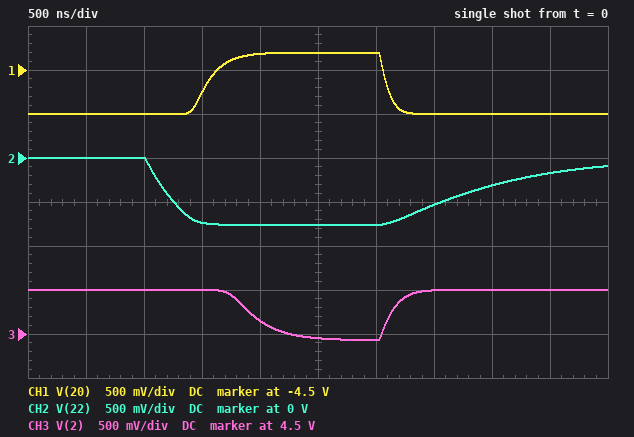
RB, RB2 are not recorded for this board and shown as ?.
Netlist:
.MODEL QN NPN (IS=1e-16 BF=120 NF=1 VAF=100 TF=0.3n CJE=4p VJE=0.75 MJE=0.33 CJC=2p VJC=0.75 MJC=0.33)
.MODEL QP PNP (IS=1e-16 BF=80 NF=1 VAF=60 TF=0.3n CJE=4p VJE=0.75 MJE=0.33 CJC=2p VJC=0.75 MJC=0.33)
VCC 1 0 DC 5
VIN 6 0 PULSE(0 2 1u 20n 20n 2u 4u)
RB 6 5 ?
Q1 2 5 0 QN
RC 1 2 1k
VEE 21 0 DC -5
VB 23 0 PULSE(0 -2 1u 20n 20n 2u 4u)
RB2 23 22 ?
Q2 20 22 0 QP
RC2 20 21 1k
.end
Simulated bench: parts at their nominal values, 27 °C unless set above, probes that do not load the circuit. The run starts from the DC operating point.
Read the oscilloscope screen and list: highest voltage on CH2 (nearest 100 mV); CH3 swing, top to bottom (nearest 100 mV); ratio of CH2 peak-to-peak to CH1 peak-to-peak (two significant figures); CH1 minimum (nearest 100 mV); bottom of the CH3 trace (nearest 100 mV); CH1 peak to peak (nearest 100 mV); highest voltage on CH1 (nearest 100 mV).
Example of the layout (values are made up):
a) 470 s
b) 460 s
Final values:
a) 0 V
b) 600 mV
c) 1.1
d) -5.0 V
e) 4.4 V
f) 700 mV
g) -4.3 V
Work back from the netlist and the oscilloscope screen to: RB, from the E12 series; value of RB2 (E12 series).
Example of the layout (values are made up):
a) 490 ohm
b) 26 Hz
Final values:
a) 270 kΩ
b) 150 kΩ
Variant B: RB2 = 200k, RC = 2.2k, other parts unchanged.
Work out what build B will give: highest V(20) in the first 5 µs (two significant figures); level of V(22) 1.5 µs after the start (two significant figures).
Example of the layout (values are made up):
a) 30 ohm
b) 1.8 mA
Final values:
a) -4.5 V
b) -660 mV
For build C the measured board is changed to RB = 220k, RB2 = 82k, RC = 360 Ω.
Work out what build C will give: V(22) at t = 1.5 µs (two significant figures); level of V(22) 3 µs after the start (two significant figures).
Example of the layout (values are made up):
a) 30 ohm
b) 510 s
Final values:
a) -770 mV
b) -780 mV
